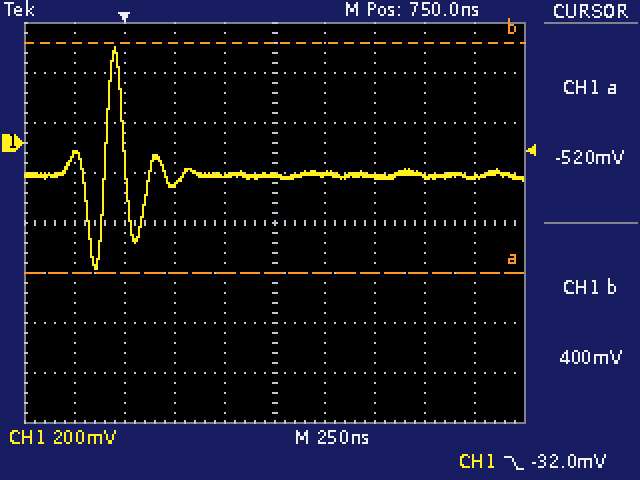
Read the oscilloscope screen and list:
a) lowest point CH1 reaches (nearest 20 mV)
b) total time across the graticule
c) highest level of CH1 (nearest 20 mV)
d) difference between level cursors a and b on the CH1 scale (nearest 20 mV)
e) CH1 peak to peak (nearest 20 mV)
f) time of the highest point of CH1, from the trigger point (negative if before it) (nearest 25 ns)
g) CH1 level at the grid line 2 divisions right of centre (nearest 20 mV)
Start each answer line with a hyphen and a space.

- -500 mV
- 2.5 µs
- 380 mV
- 920 mV
- 880 mV
- -50 ns
- -140 mV
